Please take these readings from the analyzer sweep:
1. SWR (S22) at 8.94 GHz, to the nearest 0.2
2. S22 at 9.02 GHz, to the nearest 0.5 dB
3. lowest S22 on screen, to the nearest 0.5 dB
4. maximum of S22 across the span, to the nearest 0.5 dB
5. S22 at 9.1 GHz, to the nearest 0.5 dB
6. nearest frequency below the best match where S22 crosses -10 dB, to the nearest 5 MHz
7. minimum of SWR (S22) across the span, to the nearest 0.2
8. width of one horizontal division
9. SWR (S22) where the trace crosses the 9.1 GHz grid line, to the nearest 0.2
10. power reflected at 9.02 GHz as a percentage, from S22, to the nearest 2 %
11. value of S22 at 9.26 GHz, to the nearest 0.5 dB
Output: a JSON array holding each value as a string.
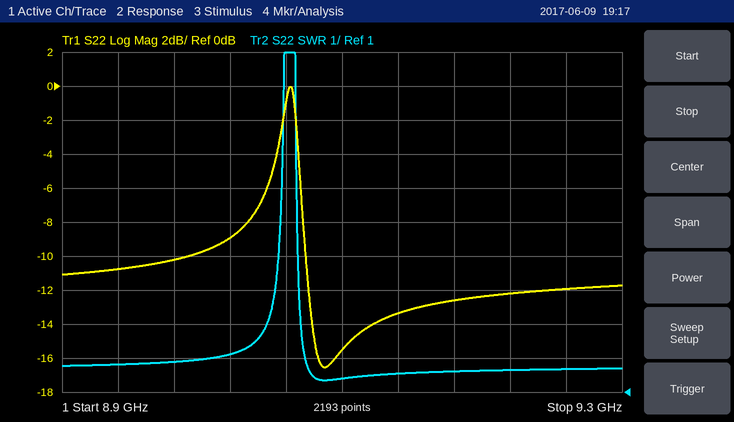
["1.8", "-9.0 dB", "-16.5 dB", "0.0 dB", "-15.5 dB", "9.075 GHz", "1.4", "40 MHz", "1.4", "12 %", "-12.0 dB"]
